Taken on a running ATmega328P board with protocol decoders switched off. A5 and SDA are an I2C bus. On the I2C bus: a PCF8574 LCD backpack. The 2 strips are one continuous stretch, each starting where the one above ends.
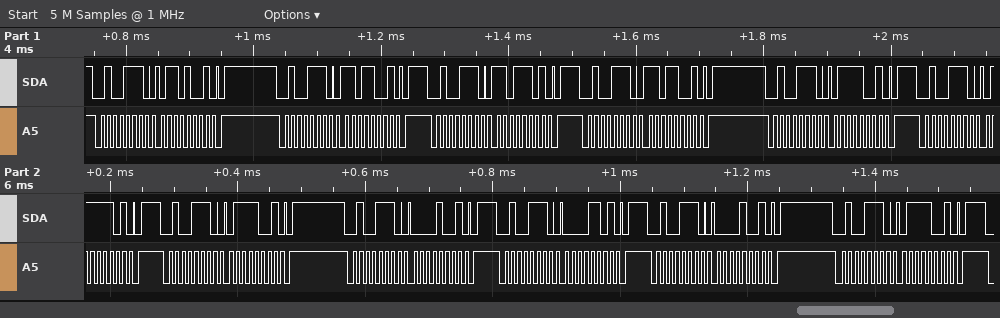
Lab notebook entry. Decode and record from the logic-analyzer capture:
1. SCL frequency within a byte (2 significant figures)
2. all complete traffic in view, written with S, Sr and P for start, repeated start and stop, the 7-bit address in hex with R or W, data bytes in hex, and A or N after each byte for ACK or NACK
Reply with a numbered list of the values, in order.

1. 100 kHz
2. S 27W A 69 A P S 27W A D9 A P S 27W A DD A P S 27W A D9 A P S 27W A 79 A P S 27W A 7D A P S 27W A 79 A P S 27W A 09 A P S 27W A 0D A P S 27W A 09 A P S 27W A 79 A P
